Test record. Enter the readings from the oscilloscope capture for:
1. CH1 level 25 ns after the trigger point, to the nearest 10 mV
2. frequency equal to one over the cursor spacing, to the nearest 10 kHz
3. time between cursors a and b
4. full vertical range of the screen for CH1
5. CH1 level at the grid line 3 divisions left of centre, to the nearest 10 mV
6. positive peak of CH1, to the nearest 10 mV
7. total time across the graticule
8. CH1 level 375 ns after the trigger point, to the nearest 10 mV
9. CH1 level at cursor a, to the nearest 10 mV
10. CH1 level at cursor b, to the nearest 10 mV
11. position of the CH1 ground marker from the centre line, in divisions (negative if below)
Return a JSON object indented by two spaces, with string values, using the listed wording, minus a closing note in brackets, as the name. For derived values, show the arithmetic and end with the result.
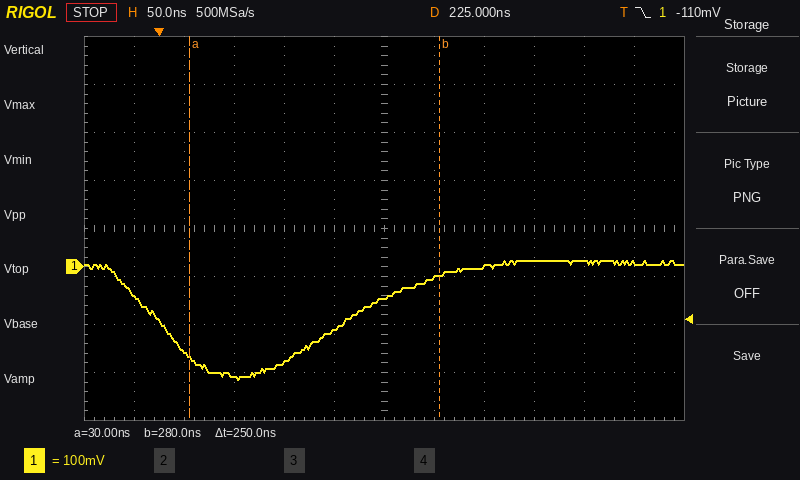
{
  "CH1 level 25 ns after the trigger point, to the nearest 10 mV": "-180 mV",
  "frequency equal to one over the cursor spacing, to the nearest 10 kHz": "1 / 250 ns ≈ 4.00 MHz",
  "time between cursors a and b": "250 ns",
  "full vertical range of the screen for CH1": "800 mV",
  "CH1 level at the grid line 3 divisions left of centre, to the nearest 10 mV": "-230 mV",
  "positive peak of CH1, to the nearest 10 mV": "10 mV",
  "total time across the graticule": "600 ns",
  "CH1 level 375 ns after the trigger point, to the nearest 10 mV": "10 mV",
  "CH1 level at cursor a, to the nearest 10 mV": "-190 mV",
  "CH1 level at cursor b, to the nearest 10 mV": "-20 mV",
  "position of the CH1 ground marker from the centre line, in divisions": "-0.8 div"
}
